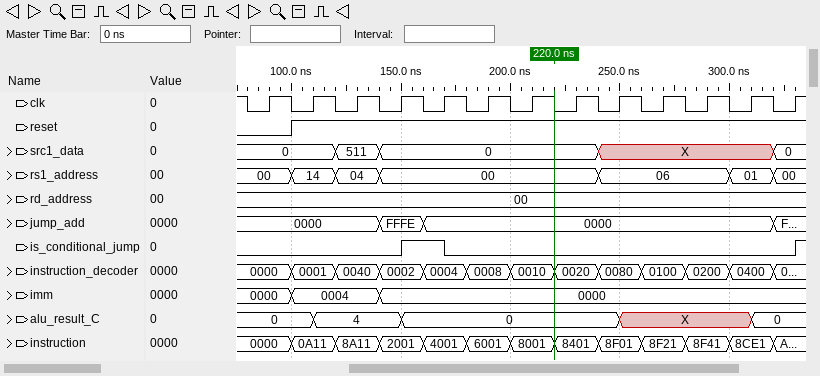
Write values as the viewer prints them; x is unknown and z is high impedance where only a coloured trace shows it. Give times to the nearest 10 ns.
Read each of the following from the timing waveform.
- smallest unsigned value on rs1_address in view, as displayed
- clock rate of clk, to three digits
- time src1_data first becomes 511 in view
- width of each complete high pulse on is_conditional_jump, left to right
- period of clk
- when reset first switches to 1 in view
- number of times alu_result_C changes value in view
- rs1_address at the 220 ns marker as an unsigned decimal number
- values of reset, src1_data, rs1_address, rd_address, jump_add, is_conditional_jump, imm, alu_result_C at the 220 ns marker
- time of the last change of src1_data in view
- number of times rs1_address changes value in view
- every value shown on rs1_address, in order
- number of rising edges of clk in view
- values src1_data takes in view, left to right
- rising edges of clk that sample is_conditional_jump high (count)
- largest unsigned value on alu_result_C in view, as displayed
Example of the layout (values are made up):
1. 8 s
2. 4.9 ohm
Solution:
1. 00
2. 50.0 MHz
3. 120 ns
4. 20 ns
5. 20 ns
6. 100 ns
7. 4
8. 0
9. reset=1, src1_data=0, rs1_address=00, rd_address=00, jump_add=0000, is_conditional_jump=0, imm=0000, alu_result_C=0
10. 320 ns
11. 6
12. 00, 14, 04, 00, 06, 01, 00
13. 13
14. 0, 511, 0, X, 0
15. 1
16. 4
